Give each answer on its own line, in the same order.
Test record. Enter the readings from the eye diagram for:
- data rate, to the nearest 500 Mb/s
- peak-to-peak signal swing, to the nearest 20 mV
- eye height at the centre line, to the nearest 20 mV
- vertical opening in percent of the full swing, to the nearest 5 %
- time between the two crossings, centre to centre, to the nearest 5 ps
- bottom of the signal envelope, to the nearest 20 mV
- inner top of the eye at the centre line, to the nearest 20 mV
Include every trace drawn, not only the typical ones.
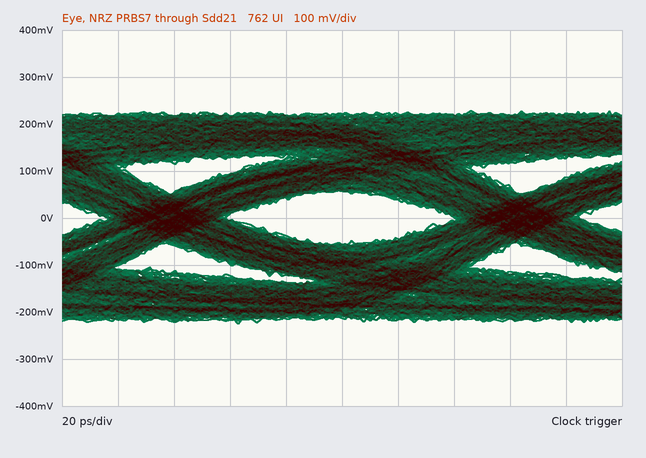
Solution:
8.0 Gb/s
460 mV
120 mV
25 %
125 ps
-220 mV
60 mV
